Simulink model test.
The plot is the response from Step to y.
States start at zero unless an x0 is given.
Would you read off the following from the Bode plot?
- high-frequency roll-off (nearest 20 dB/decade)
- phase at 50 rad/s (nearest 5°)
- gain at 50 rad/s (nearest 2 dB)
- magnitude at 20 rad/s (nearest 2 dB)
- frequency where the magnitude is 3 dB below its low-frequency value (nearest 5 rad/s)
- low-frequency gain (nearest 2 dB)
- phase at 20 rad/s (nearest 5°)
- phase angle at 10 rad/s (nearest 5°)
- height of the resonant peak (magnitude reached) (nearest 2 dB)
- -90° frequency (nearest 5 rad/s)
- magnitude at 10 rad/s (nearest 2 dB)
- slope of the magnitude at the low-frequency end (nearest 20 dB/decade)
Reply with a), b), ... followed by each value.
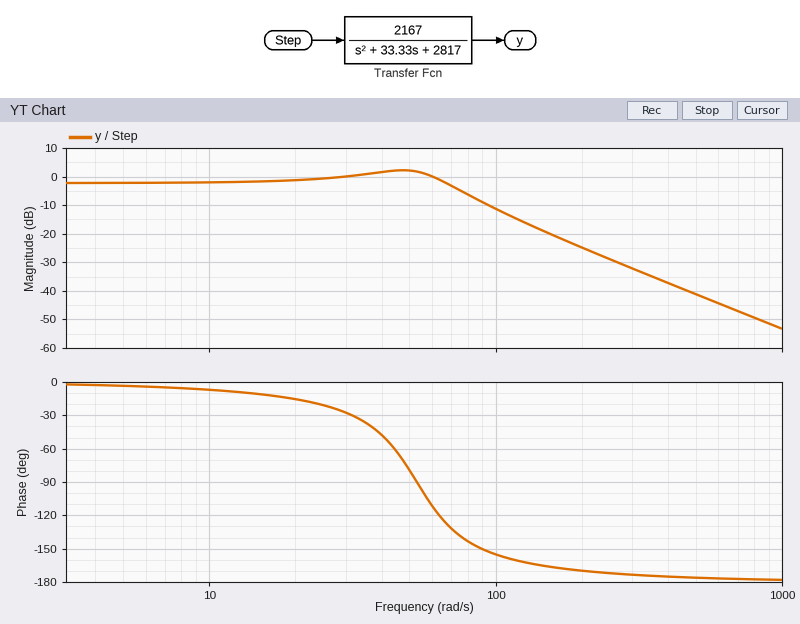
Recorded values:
a) -40 dB/decade
b) -80°
c) 2 dB
d) -2 dB
e) 75 rad/s
f) -2 dB
g) -15°
h) -5°
i) 2 dB
j) 55 rad/s
k) -2 dB
l) 0 dB/decade
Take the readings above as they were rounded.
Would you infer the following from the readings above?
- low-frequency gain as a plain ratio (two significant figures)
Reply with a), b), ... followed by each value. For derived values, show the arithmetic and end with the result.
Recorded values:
a) 10^(-2 / 20) = 0.79
